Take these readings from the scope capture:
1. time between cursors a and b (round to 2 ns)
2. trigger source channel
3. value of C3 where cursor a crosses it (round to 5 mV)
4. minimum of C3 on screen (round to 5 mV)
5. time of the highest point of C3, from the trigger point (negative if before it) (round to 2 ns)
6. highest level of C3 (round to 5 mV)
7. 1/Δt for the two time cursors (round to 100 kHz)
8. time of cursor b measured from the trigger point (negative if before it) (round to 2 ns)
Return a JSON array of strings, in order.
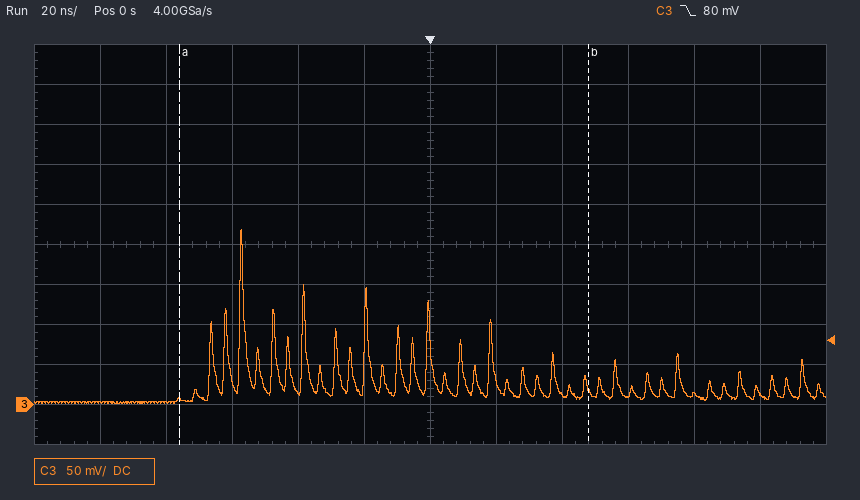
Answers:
["124 ns", "C3", "5 mV", "0 mV", "-58 ns", "220 mV", "8.1 MHz", "+48 ns"]
